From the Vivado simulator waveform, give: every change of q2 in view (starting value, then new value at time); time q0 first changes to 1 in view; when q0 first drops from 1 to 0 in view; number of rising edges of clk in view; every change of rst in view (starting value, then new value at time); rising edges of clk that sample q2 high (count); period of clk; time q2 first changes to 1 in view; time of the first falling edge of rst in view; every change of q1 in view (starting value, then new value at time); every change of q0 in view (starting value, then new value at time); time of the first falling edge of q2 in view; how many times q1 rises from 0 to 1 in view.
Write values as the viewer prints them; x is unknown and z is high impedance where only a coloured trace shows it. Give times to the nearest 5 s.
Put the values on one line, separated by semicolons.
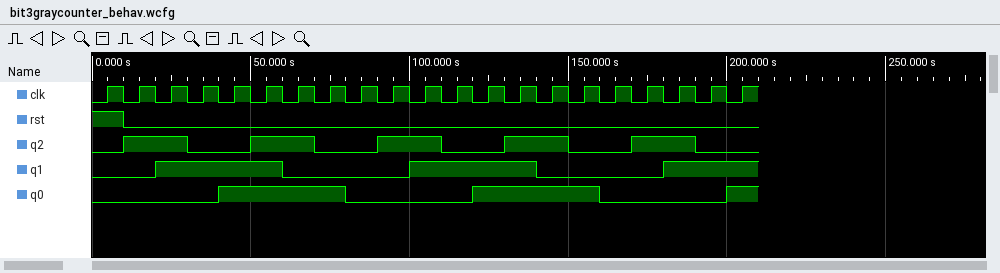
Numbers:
0, 1 at 10 s, 0 at 30 s, 1 at 50 s, 0 at 70 s, 1 at 90 s, 0 at 110 s, 1 at 130 s, 0 at 150 s, 1 at 170 s, 0 at 190 s; 40 s; 80 s; 21; 1, 0 at 10 s; 10; 10 s; 10 s; 10 s; 0, 1 at 20 s, 0 at 60 s, 1 at 100 s, 0 at 140 s, 1 at 180 s; 0, 1 at 40 s, 0 at 80 s, 1 at 120 s, 0 at 160 s, 1 at 200 s; 30 s; 3
